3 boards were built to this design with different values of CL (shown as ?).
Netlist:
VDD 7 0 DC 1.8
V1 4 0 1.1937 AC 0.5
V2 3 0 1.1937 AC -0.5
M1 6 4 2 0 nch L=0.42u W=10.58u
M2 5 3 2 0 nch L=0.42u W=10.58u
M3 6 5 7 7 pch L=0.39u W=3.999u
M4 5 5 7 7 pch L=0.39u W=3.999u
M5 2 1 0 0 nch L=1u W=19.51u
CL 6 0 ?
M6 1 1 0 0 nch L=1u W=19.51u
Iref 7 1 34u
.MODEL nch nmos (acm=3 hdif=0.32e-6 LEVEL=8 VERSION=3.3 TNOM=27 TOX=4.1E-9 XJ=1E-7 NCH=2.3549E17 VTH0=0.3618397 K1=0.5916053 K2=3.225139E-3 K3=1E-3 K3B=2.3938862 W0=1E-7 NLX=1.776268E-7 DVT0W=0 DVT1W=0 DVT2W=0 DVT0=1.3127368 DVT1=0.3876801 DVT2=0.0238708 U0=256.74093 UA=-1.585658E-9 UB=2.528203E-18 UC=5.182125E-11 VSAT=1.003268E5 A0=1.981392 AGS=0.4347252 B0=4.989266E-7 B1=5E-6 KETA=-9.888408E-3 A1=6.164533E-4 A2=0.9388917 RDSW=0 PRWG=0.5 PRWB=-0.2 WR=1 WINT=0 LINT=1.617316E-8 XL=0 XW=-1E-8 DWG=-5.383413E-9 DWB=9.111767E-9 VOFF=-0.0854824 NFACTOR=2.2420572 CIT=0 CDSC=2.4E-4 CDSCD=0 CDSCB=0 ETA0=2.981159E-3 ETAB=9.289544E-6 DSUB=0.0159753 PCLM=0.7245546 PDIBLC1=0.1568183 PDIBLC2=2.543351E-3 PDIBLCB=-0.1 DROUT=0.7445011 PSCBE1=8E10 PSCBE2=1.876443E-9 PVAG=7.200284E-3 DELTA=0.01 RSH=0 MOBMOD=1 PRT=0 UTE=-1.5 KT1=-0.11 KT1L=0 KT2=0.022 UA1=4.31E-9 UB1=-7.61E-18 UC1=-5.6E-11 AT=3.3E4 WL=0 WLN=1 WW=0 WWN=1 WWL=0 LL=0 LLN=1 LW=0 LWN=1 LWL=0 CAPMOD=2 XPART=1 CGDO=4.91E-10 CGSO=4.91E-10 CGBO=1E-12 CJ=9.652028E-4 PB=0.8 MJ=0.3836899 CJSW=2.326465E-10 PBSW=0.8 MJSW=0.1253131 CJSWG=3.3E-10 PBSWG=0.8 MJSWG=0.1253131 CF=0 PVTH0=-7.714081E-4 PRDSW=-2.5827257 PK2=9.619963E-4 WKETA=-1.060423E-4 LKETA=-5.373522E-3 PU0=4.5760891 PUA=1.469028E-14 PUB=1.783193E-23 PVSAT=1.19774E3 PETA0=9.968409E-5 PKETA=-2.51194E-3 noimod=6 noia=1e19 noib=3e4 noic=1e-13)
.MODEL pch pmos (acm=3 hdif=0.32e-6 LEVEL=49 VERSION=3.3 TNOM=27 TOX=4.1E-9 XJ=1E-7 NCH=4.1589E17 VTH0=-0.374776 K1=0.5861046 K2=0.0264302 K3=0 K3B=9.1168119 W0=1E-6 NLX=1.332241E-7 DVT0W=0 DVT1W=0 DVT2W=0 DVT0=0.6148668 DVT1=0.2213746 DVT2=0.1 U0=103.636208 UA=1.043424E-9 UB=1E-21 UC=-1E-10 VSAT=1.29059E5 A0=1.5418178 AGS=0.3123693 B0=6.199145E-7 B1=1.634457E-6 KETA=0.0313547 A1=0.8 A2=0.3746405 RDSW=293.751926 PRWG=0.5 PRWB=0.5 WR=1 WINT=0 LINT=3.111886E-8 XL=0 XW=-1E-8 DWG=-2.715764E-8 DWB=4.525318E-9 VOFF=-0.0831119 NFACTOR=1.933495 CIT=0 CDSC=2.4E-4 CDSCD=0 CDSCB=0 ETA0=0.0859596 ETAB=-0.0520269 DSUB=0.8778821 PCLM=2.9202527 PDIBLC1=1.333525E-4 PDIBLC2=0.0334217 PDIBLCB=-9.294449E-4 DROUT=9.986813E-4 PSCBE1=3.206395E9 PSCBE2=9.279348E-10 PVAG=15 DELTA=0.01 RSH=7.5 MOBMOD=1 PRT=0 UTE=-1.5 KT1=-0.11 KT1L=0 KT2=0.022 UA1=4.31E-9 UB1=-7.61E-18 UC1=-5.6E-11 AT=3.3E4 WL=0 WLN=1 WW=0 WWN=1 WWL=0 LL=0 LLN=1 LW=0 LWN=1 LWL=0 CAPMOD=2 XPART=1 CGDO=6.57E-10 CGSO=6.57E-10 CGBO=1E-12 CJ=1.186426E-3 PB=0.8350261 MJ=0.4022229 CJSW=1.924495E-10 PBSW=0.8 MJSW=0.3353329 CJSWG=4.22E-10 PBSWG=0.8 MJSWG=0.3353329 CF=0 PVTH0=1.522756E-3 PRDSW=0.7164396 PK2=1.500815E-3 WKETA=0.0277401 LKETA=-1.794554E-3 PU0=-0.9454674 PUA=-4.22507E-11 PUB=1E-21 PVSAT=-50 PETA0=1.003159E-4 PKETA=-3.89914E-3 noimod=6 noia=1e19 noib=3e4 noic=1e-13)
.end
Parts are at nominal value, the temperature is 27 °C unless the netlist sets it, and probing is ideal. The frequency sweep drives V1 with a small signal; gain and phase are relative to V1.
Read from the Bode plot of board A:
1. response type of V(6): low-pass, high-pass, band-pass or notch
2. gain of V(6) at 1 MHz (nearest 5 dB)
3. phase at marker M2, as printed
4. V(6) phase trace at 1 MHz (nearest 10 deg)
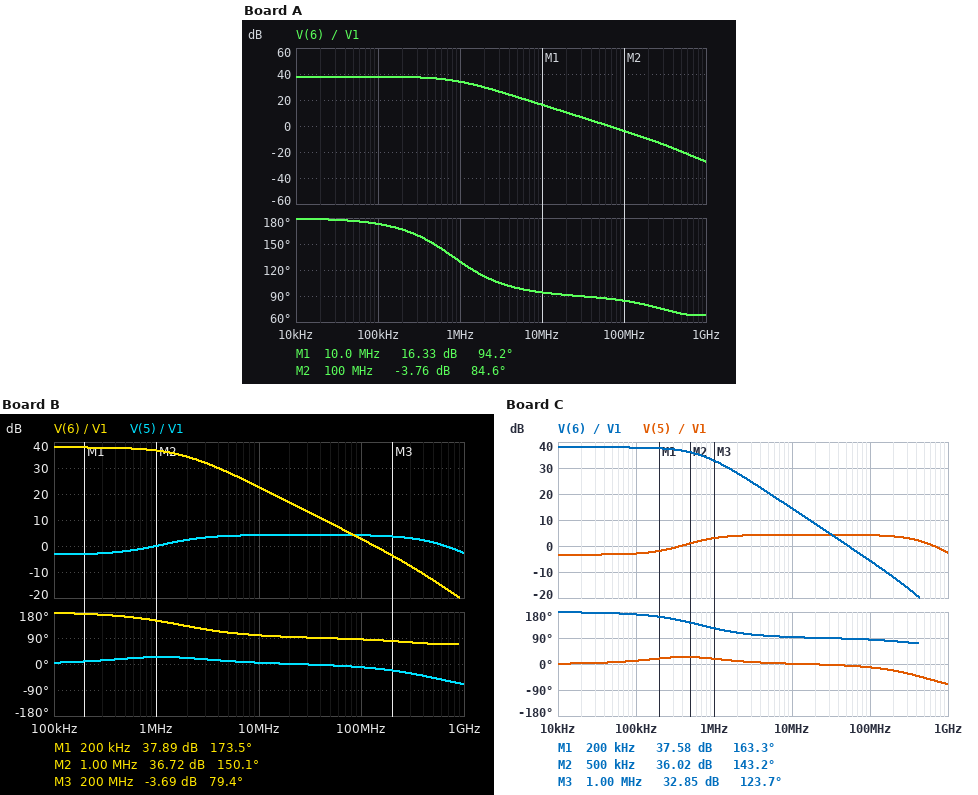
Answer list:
low-pass
35 dB
84.6 deg
130 deg
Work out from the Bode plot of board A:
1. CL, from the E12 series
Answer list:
1.2 pF
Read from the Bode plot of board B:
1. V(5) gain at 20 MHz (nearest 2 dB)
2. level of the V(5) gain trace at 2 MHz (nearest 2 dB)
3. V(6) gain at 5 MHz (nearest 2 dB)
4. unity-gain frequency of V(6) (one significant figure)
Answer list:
4 dB
2 dB
28 dB
100 MHz
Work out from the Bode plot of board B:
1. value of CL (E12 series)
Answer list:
560 fF
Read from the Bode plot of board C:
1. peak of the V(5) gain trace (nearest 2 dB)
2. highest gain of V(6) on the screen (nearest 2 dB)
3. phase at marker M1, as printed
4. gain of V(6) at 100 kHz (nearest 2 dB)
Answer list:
4 dB
38 dB
163.3 deg
38 dB
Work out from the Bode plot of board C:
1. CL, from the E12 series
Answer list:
1.5 pF
